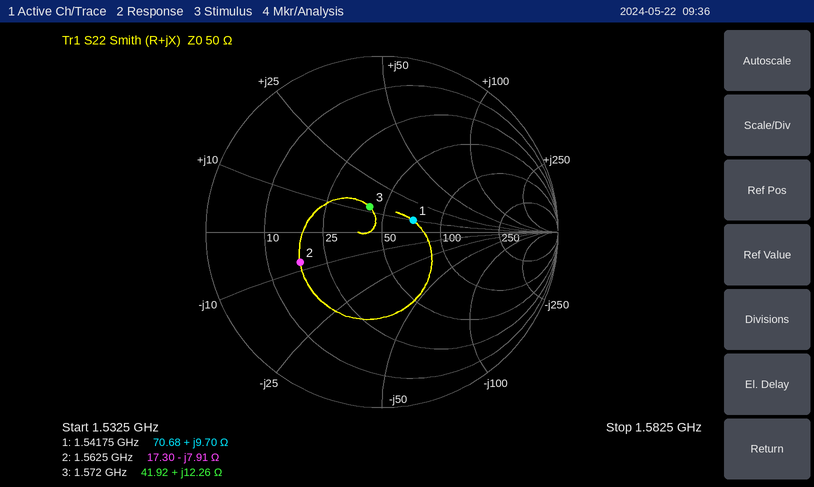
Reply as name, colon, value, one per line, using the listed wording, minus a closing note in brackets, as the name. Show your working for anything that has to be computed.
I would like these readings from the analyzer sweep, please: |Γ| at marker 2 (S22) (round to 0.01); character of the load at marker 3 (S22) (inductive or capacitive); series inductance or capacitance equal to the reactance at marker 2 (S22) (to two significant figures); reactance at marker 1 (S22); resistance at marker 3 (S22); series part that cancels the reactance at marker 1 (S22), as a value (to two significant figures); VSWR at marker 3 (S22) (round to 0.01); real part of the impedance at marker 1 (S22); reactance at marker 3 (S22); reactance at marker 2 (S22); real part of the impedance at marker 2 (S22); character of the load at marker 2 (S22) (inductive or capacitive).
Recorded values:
|Γ| at marker 2 (S22): 0.50
character of the load at marker 3 (S22): inductive
series inductance or capacitance equal to the reactance at marker 2 (S22): C = 1/(2π × 1.5625 GHz × 7.91 Ω) ≈ 13 pF
reactance at marker 1: +9.70 Ω
resistance at marker 3: 41.92 Ω
series part that cancels the reactance at marker 1 (S22), as a value: C = 1/(2π × 1.54175 GHz × 9.7 Ω) ≈ 11 pF
VSWR at marker 3 (S22): 1.38
real part of the impedance at marker 1: 70.68 Ω
reactance at marker 3: +12.26 Ω
reactance at marker 2: -7.91 Ω
real part of the impedance at marker 2: 17.30 Ω
character of the load at marker 2 (S22): capacitive
